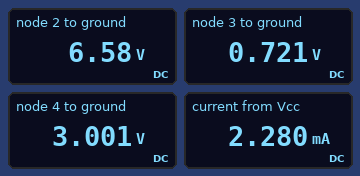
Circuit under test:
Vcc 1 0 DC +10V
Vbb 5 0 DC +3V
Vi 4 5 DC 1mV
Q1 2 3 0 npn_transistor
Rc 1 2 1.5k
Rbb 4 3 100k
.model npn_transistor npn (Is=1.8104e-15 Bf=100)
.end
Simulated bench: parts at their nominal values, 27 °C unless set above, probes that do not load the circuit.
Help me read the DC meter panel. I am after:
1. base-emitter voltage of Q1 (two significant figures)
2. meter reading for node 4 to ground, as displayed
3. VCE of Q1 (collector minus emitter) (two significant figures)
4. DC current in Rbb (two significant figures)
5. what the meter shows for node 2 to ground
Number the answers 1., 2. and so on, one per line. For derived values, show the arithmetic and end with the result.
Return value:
1. 721 mV = 720 mV
2. 3.001 V
3. 6.58 V = 6.6 V
4. (3.001 V - 721 mV) / 100 kΩ = 23 µA
5. 6.58 V
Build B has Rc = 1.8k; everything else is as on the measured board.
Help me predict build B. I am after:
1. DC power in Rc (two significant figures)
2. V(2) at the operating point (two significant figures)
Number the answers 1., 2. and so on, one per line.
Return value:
1. 9.4 mW
2. 5.9 V
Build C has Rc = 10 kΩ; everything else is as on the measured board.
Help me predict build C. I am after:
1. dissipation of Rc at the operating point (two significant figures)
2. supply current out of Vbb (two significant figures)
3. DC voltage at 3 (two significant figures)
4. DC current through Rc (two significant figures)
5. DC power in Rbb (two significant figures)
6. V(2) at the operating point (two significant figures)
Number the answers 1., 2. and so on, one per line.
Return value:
1. 9.8 mW
2. 23 µA
3. 700 mV
4. 990 µA
5. 53 µW
6. 110 mV
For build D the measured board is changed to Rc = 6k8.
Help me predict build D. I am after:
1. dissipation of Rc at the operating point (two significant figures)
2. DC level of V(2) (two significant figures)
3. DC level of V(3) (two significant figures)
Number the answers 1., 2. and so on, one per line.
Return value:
1. 14 mW
2. 130 mV
3. 710 mV
